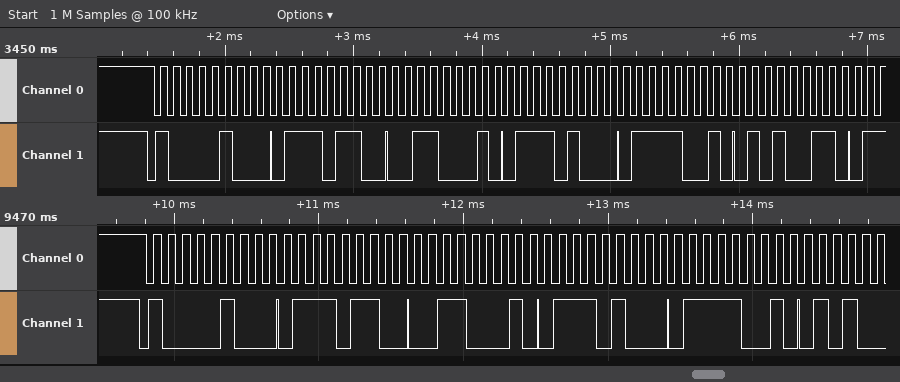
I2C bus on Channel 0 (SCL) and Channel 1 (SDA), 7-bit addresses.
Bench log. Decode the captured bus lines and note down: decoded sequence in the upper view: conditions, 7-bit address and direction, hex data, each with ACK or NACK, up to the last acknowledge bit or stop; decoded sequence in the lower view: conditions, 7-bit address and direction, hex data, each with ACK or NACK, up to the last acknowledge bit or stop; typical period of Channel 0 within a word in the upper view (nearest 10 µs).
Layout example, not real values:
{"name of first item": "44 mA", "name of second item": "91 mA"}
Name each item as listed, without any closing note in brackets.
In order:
{"decoded sequence in the upper view: conditions, 7-bit address and direction, hex data, each with ACK or NACK, up to the last acknowledge bit or stop": "start, address 42 write ACK, 76 ACK, 31 ACK, 74 ACK, 79 ACK, 53 ACK", "decoded sequence in the lower view: conditions, 7-bit address and direction, hex data, each with ACK or NACK, up to the last acknowledge bit or stop": "start, address 42 write ACK, 76 ACK, 31 ACK, 74 ACK, 79 ACK", "typical period of Channel 0 within a word in the upper view": "100 µs"}
